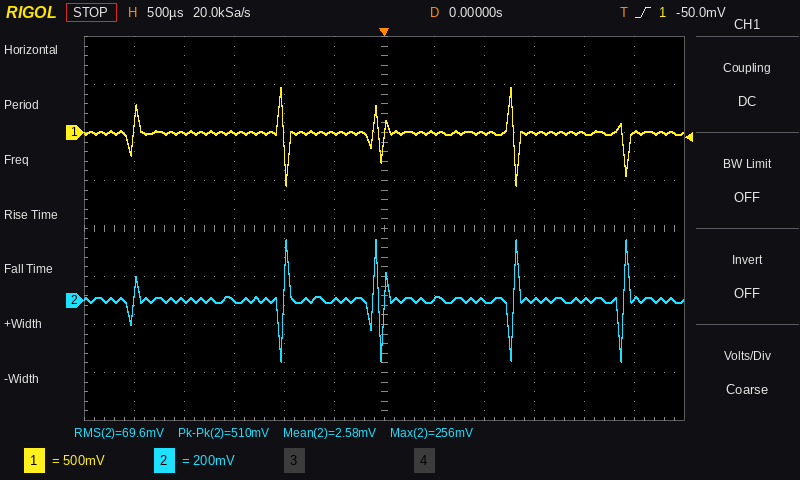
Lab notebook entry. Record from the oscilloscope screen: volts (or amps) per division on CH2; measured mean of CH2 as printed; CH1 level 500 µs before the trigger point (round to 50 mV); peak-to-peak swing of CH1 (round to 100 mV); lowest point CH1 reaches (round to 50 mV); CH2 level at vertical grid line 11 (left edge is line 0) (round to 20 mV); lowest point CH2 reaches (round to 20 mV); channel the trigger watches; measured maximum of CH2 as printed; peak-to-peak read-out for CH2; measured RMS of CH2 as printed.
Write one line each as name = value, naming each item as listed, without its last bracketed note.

volts (or amps) per division on CH2 = 200 mV
measured mean of CH2 as printed = 2.58 mV
CH1 level 500 µs before the trigger point = 0 mV
peak-to-peak swing of CH1 = 1.00 V
lowest point CH1 reaches = -550 mV
CH2 level at vertical grid line 11 (left edge is line 0) = 0 mV
lowest point CH2 reaches = -260 mV
channel the trigger watches = CH1
measured maximum of CH2 as printed = 256 mV
peak-to-peak read-out for CH2 = 510 mV
measured RMS of CH2 as printed = 69.6 mV
